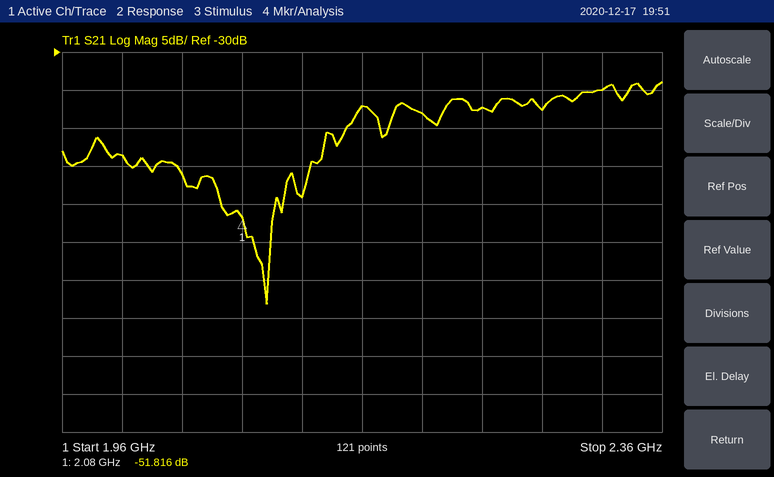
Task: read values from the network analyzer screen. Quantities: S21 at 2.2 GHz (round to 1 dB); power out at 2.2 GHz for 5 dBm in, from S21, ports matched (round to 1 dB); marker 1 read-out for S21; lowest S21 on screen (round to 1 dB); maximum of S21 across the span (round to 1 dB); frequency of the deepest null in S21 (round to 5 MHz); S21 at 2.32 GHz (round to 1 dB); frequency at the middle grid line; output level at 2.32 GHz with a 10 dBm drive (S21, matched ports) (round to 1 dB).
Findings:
-38 dB
-33 dBm
-51.816 dB
-63 dB
-34 dB
2.095 GHz
-35 dB
2.16 GHz
-25 dBm
